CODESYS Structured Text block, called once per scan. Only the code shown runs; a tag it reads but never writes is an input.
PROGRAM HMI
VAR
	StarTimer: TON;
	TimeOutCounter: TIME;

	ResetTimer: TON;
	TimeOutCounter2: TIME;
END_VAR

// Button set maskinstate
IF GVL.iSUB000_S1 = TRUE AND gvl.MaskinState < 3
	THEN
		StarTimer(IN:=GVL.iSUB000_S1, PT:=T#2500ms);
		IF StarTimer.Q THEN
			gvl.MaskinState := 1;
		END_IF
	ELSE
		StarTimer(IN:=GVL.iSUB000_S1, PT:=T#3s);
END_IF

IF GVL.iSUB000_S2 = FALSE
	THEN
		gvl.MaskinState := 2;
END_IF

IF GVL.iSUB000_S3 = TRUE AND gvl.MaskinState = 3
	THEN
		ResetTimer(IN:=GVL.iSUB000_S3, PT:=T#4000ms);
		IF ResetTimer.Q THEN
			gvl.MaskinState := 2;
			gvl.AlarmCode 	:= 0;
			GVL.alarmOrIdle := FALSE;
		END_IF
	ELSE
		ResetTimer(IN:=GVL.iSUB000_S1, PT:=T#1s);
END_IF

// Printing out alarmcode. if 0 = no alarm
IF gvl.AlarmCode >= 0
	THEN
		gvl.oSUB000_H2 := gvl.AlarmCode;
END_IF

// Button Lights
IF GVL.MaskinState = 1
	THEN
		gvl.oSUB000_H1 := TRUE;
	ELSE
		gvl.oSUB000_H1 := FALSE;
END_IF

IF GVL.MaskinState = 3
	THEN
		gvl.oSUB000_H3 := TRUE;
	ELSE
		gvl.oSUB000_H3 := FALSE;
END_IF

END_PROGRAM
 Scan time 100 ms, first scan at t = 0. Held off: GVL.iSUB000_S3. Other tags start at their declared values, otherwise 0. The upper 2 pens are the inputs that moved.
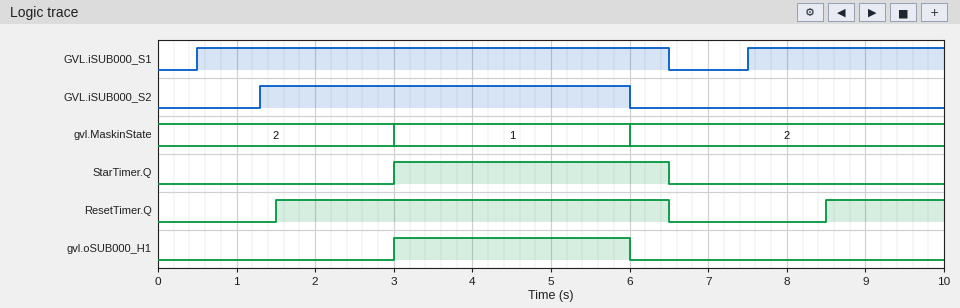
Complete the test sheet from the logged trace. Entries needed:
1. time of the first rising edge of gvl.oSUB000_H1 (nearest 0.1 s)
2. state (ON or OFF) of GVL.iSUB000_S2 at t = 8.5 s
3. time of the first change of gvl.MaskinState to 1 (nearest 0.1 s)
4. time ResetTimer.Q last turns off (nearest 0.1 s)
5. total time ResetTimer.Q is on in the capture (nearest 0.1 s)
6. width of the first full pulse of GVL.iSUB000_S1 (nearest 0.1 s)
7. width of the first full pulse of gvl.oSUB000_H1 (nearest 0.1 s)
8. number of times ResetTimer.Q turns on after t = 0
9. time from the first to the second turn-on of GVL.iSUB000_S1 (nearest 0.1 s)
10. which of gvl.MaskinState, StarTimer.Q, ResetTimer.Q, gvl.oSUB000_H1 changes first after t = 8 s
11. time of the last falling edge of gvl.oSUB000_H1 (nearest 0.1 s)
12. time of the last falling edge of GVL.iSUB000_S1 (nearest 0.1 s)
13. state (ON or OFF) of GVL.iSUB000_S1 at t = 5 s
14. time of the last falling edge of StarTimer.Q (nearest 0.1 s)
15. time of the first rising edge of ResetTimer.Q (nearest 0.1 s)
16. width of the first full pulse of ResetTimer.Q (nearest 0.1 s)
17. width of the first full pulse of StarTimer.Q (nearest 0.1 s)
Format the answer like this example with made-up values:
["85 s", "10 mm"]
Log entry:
["3.0 s", "OFF", "3.0 s", "6.5 s", "6.5 s", "6.0 s", "3.0 s", "2", "7.0 s", "ResetTimer.Q", "6.0 s", "6.5 s", "ON", "6.5 s", "1.5 s", "5.0 s", "3.5 s"]
